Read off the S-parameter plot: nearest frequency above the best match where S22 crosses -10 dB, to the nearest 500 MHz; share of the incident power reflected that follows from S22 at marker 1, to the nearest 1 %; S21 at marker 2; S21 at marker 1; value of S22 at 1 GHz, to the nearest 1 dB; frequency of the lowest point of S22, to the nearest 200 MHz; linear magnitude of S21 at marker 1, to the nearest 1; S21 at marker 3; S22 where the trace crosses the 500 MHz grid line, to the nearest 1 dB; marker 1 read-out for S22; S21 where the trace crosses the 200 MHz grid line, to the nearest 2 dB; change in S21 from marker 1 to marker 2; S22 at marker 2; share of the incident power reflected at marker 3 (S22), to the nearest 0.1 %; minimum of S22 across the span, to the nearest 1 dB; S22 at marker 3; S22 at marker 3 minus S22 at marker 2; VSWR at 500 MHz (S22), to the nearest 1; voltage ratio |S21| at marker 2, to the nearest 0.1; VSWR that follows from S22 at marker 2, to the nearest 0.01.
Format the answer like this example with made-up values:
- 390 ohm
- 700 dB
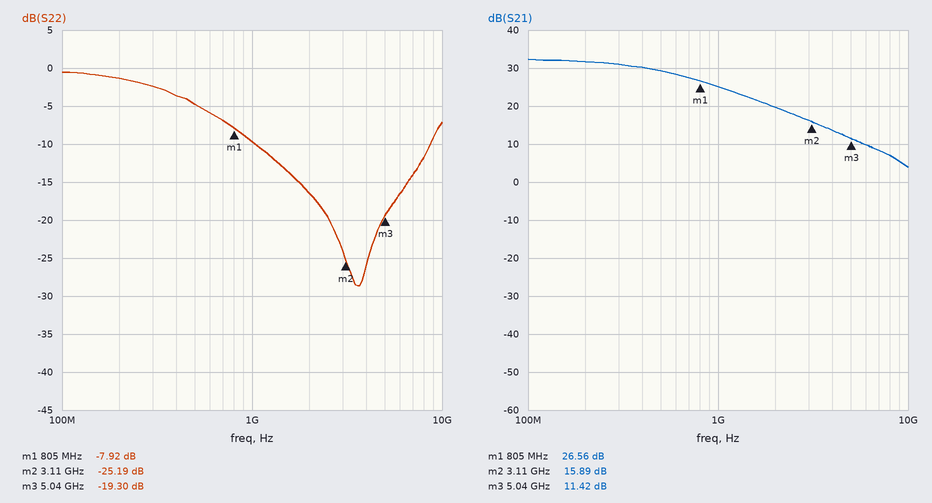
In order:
- 8.5 GHz
- 16 %
- 15.89 dB
- 26.56 dB
- -10 dB
- 3.6 GHz
- 21
- 11.42 dB
- -5 dB
- -7.92 dB
- 32 dB
- -10.67 dB
- -25.19 dB
- 1.2 %
- -29 dB
- -19.30 dB
- 5.89 dB
- 4
- 6.2
- 1.12
